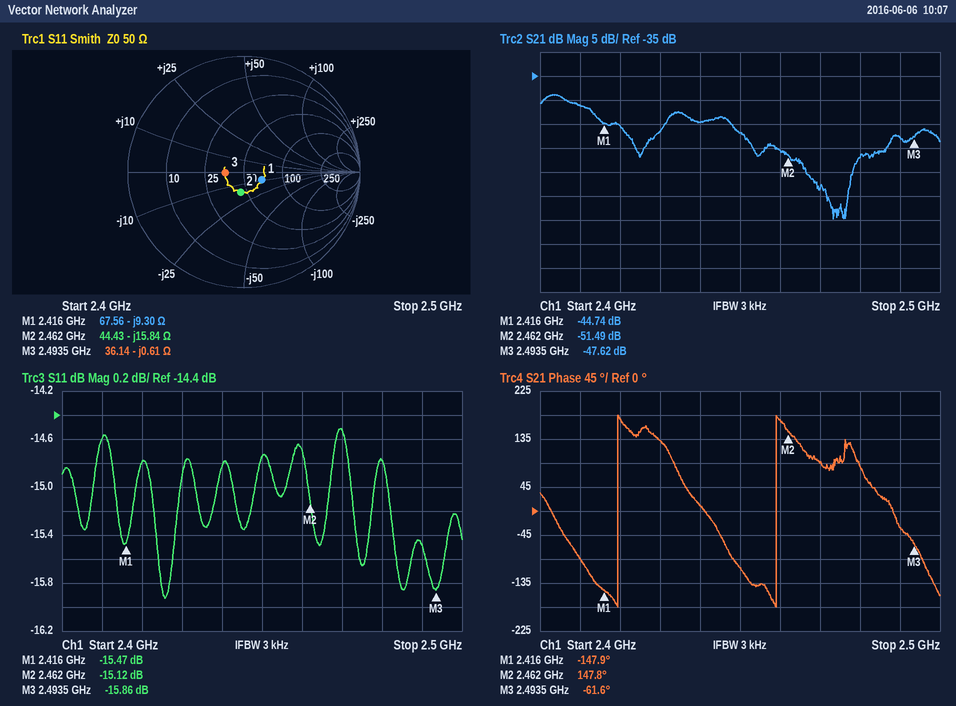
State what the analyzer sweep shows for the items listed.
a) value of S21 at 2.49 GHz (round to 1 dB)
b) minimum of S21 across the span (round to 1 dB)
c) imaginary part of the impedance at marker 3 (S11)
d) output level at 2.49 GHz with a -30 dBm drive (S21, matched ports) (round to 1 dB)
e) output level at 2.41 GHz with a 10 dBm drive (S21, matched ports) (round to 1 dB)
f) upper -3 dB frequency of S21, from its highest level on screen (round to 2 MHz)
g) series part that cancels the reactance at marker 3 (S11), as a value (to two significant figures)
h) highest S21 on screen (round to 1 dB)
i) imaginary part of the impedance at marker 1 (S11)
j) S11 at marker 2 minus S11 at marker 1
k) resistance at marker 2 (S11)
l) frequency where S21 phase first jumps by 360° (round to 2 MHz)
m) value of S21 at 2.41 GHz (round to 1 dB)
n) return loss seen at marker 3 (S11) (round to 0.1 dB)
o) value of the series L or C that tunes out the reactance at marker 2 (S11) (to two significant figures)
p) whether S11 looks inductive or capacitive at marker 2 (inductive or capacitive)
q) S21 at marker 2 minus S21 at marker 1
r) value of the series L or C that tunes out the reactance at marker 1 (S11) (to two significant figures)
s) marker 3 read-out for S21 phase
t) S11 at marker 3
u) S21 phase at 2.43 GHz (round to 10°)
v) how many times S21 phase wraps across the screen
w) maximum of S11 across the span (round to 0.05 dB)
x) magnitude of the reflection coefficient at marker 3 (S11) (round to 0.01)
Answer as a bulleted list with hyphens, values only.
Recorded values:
- -48 dB
- -65 dB
- -0.61 Ω
- -78 dBm
- -31 dBm
- 2.412 GHz
- 39 pH
- -39 dB
- -9.30 Ω
- 0.35 dB
- 44.43 Ω
- 2.420 GHz
- -41 dB
- 15.9 dB
- 1.0 nH
- capacitive
- -6.75 dB
- 610 pH
- -61.6°
- -15.86 dB
- 130°
- 2
- -14.50 dB
- 0.16
